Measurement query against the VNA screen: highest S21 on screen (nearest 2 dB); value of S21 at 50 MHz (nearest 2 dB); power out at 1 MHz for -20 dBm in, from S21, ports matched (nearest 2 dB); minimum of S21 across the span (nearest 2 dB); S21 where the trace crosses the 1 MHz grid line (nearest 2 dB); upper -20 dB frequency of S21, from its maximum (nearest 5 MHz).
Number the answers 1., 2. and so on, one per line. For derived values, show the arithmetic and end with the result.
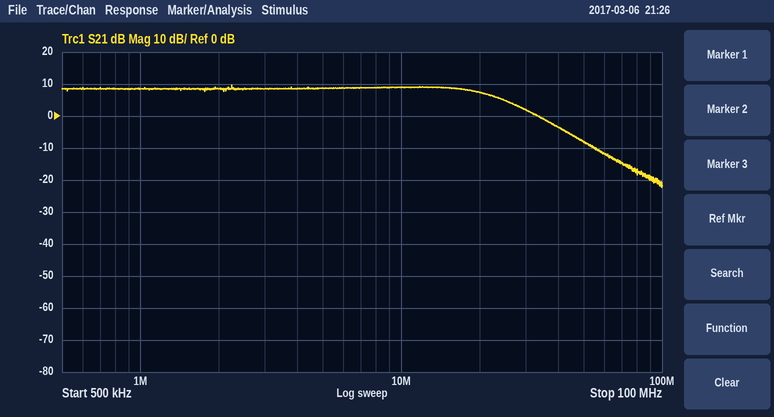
1. 10 dB
2. -8 dB
3. -20 dBm + (8 dB) = -12 dBm
4. -22 dB
5. 8 dB
6. 55 MHz
